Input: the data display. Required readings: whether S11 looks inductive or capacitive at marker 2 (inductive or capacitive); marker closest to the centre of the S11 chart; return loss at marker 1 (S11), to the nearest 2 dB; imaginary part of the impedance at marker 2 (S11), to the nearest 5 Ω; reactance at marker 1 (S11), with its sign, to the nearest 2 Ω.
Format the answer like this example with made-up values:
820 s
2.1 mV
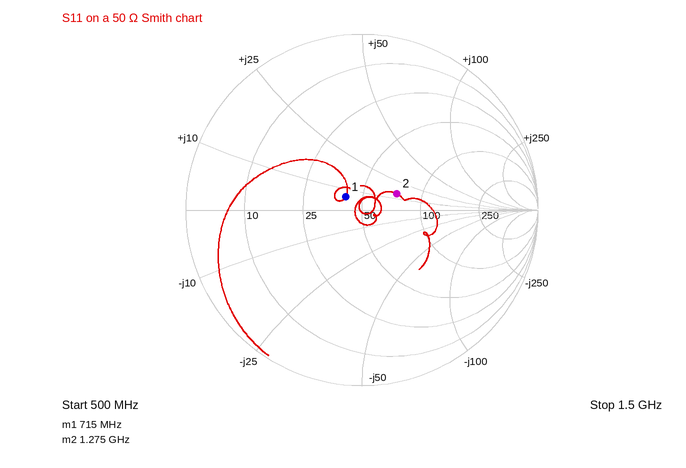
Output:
inductive
marker 1
18 dB
+15 Ω
+6 Ω
